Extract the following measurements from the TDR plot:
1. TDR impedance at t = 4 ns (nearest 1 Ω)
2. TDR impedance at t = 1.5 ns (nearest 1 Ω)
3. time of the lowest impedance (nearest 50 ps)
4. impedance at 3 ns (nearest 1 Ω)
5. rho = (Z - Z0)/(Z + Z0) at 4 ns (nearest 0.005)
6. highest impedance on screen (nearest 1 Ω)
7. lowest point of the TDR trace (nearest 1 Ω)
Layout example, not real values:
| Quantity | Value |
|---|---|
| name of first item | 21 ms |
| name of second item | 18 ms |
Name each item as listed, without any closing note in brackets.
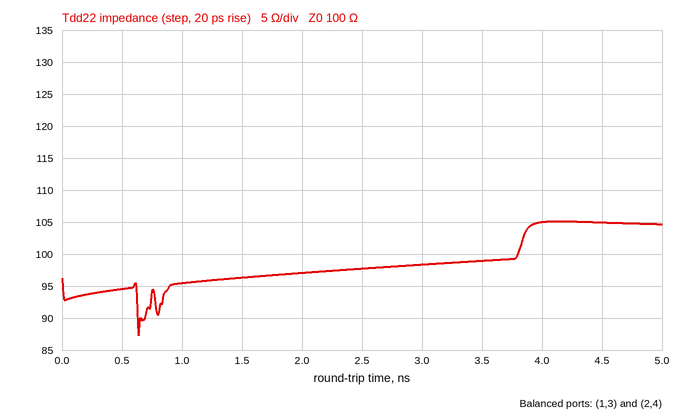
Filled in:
| Quantity | Value |
|---|---|
| TDR impedance at t = 4 ns | 105 Ω |
| TDR impedance at t = 1.5 ns | 96 Ω |
| time of the lowest impedance | 650 ps |
| impedance at 3 ns | 98 Ω |
| rho = (Z - Z0)/(Z + Z0) at 4 ns | +0.025 |
| highest impedance on screen | 105 Ω |
| lowest point of the TDR trace | 87 Ω |
